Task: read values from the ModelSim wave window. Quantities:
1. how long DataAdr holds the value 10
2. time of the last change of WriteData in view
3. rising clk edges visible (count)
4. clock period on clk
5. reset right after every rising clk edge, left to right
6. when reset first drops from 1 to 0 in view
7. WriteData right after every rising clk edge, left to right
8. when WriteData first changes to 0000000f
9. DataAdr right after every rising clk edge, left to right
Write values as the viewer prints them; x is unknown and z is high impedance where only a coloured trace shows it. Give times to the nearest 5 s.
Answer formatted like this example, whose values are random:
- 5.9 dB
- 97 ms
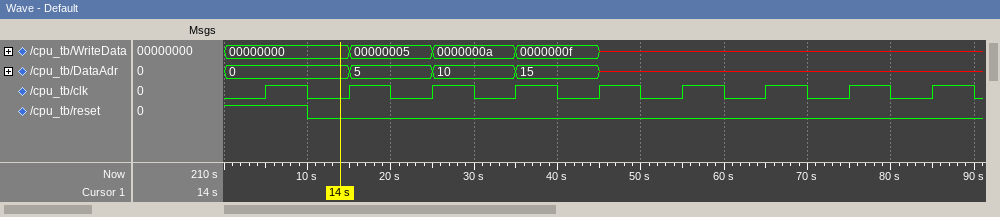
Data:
- 10 s
- 45 s
- 9
- 10 s
- 1 0 0 0 0 0 0 0 0
- 10 s
- 00000000, 00000005, 0000000a, 0000000f, x, x, x, x, x
- 35 s
- 0, 5, 10, 15, x, x, x, x, x
